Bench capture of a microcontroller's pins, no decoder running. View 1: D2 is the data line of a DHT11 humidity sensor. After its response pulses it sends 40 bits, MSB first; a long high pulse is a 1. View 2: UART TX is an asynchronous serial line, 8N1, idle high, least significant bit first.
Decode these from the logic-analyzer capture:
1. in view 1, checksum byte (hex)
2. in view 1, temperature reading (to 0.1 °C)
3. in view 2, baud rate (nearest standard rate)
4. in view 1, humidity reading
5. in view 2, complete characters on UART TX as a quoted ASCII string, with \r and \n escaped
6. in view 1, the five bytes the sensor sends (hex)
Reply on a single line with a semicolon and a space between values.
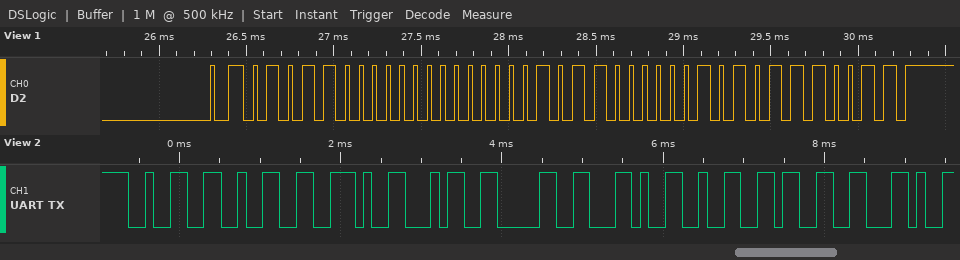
0x73; 22.5 °C; 9600 baud; 88 %; "22.40,23,"; 58 00 16 05 73
